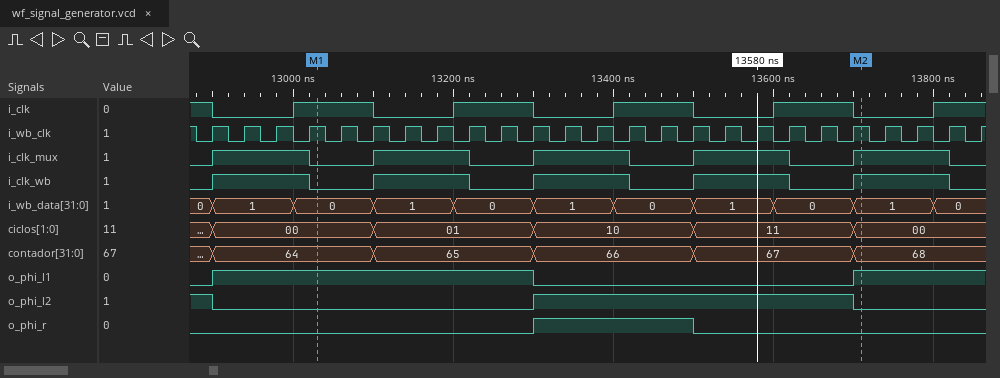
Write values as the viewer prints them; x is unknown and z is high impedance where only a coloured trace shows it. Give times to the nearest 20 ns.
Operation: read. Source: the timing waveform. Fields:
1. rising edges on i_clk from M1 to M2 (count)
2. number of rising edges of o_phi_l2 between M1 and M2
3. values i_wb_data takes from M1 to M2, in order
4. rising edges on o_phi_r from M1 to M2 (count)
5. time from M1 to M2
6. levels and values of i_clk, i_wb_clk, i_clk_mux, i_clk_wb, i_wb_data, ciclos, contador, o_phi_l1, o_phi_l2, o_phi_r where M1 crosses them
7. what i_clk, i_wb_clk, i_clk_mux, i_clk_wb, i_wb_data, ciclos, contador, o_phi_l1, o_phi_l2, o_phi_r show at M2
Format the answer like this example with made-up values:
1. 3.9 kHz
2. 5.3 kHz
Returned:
1. 3
2. 1
3. 0, 1, 0, 1, 0, 1, 0, 1
4. 1
5. 680 ns
6. i_clk=1, i_wb_clk=1, i_clk_mux=0, i_clk_wb=0, i_wb_data=0, ciclos=00, contador=64, o_phi_l1=1, o_phi_l2=0, o_phi_r=0
7. i_clk=0, i_wb_clk=1, i_clk_mux=1, i_clk_wb=1, i_wb_data=1, ciclos=00, contador=68, o_phi_l1=1, o_phi_l2=0, o_phi_r=0
